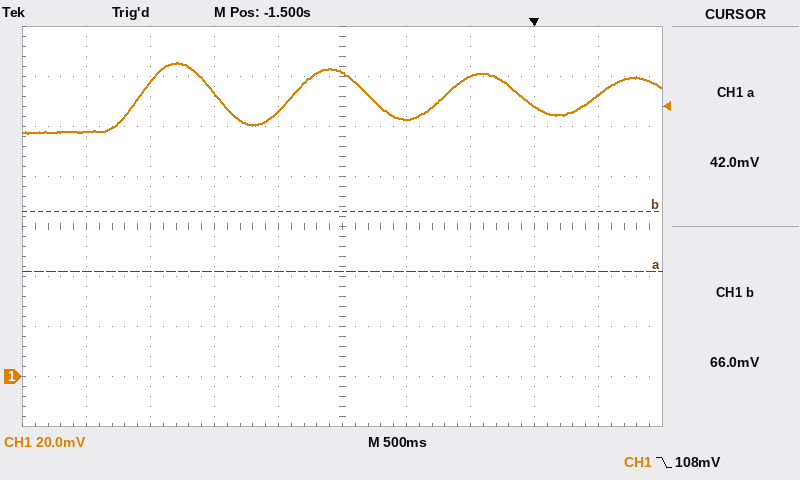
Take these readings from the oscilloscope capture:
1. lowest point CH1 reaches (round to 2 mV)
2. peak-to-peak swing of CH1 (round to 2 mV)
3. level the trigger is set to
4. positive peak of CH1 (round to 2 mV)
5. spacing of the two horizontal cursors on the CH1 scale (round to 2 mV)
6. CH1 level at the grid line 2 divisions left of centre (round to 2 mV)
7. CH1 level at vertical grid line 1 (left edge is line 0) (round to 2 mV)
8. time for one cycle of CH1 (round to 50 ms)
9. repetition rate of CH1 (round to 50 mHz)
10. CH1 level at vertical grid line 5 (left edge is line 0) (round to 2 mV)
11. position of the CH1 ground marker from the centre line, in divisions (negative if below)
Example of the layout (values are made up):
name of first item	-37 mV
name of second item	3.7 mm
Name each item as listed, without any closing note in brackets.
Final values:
lowest point CH1 reaches	98 mV
peak-to-peak swing of CH1	28 mV
level the trigger is set to	108 mV
positive peak of CH1	126 mV
spacing of the two horizontal cursors on the CH1 scale	24 mV
CH1 level at the grid line 2 divisions left of centre	114 mV
CH1 level at vertical grid line 1 (left edge is line 0)	98 mV
time for one cycle of CH1	1.20 s
repetition rate of CH1	850 mHz
CH1 level at vertical grid line 5 (left edge is line 0)	122 mV
position of the CH1 ground marker from the centre line, in divisions	-3.0 div
